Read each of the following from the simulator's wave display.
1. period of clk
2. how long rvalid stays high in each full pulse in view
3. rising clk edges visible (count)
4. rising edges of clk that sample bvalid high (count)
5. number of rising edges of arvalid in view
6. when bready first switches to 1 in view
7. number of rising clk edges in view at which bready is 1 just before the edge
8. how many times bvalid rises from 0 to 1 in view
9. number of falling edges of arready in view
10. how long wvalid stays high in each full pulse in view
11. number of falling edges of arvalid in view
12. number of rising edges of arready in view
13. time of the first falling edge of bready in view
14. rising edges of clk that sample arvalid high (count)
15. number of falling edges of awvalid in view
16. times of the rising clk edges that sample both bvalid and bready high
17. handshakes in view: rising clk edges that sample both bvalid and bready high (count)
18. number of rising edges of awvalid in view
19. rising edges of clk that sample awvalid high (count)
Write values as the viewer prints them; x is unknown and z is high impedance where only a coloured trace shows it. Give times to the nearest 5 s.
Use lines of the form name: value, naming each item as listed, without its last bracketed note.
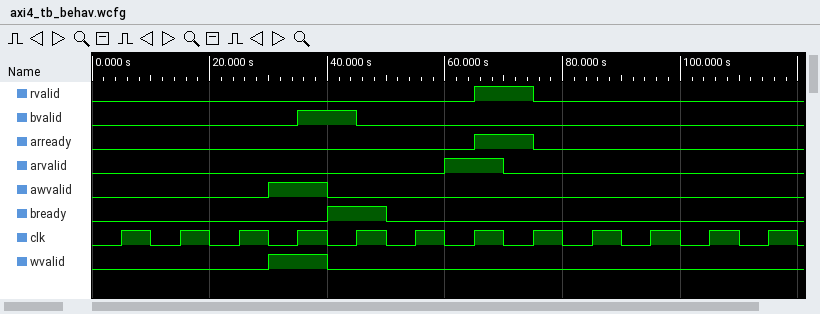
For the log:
period of clk: 10 s
how long rvalid stays high in each full pulse in view: 10 s
rising clk edges visible: 12
rising edges of clk that sample bvalid high: 1
number of rising edges of arvalid in view: 1
when bready first switches to 1 in view: 40 s
number of rising clk edges in view at which bready is 1 just before the edge: 1
how many times bvalid rises from 0 to 1 in view: 1
number of falling edges of arready in view: 1
how long wvalid stays high in each full pulse in view: 10 s
number of falling edges of arvalid in view: 1
number of rising edges of arready in view: 1
time of the first falling edge of bready in view: 50 s
rising edges of clk that sample arvalid high: 1
number of falling edges of awvalid in view: 1
times of the rising clk edges that sample both bvalid and bready high: 45 s
handshakes in view: rising clk edges that sample both bvalid and bready high: 1
number of rising edges of awvalid in view: 1
rising edges of clk that sample awvalid high: 1
